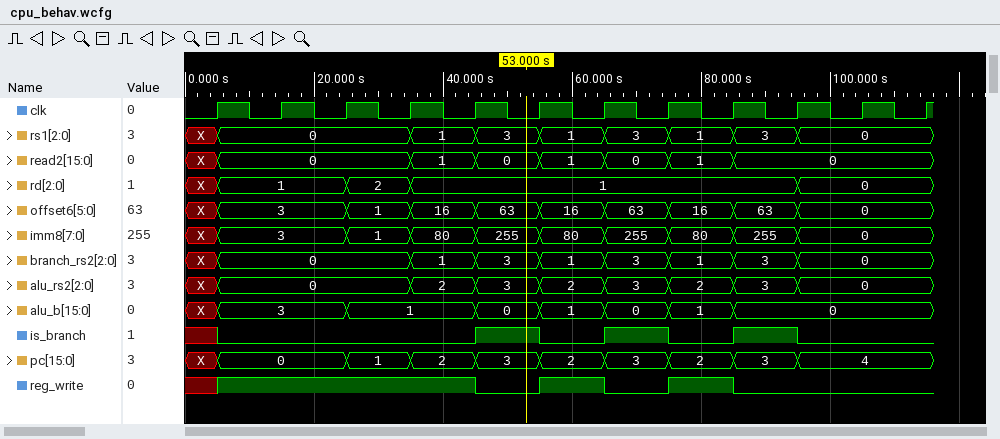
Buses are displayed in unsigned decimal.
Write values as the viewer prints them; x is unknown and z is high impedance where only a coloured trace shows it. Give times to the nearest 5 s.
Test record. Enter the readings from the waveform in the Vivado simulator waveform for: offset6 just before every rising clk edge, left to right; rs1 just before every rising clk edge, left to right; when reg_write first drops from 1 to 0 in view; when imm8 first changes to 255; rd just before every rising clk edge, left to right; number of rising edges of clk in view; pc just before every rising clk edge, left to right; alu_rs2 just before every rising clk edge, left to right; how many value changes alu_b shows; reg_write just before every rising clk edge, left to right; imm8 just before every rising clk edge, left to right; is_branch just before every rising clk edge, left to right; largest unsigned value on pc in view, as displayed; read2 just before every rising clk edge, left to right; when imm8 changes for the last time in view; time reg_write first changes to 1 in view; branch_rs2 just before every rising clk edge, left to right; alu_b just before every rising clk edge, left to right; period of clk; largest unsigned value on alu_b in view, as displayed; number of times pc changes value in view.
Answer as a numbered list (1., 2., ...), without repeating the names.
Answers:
1. X, 3, 3, 1, 16, 63, 16, 63, 16, 63, 0, 0
2. X, 0, 0, 0, 1, 3, 1, 3, 1, 3, 0, 0
3. 45 s
4. 45 s
5. X, 1, 1, 2, 1, 1, 1, 1, 1, 1, 0, 0
6. 12
7. X, 0, 0, 1, 2, 3, 2, 3, 2, 3, 4, 4
8. X, 0, 0, 0, 2, 3, 2, 3, 2, 3, 0, 0
9. 7
10. x 1 1 1 1 0 1 0 1 0 0 0
11. X, 3, 3, 1, 80, 255, 80, 255, 80, 255, 0, 0
12. x 0 0 0 0 1 0 1 0 1 0 0
13. 4
14. X, 0, 0, 0, 1, 0, 1, 0, 1, 0, 0, 0
15. 95 s
16. 5 s
17. X, 0, 0, 0, 1, 3, 1, 3, 1, 3, 0, 0
18. X, 3, 3, 1, 1, 0, 1, 0, 1, 0, 0, 0
19. 10 s
20. 3
21. 9
